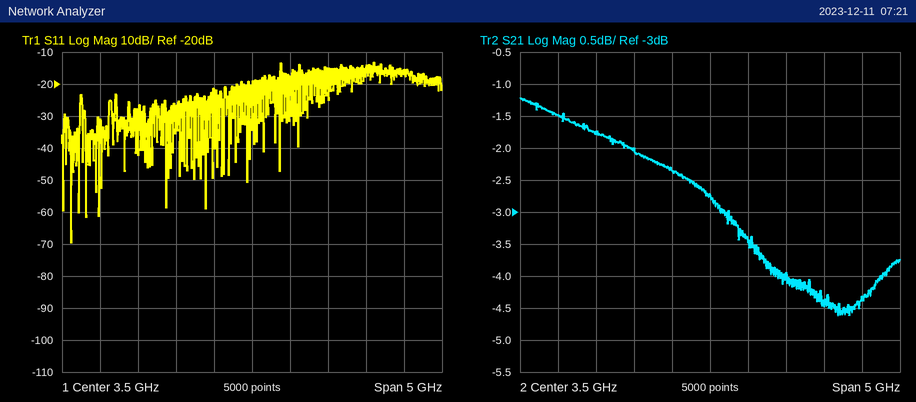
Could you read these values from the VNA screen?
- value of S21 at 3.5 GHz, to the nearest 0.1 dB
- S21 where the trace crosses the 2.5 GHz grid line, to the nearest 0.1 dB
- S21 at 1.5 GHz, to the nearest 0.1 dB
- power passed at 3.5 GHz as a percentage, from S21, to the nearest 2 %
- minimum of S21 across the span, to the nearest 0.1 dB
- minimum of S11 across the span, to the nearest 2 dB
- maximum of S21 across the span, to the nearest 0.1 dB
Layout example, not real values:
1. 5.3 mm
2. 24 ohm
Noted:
1. -2.7 dB
2. -2.0 dB
3. -1.5 dB
4. 54 %
5. -4.6 dB
6. -70 dB
7. -1.2 dB
